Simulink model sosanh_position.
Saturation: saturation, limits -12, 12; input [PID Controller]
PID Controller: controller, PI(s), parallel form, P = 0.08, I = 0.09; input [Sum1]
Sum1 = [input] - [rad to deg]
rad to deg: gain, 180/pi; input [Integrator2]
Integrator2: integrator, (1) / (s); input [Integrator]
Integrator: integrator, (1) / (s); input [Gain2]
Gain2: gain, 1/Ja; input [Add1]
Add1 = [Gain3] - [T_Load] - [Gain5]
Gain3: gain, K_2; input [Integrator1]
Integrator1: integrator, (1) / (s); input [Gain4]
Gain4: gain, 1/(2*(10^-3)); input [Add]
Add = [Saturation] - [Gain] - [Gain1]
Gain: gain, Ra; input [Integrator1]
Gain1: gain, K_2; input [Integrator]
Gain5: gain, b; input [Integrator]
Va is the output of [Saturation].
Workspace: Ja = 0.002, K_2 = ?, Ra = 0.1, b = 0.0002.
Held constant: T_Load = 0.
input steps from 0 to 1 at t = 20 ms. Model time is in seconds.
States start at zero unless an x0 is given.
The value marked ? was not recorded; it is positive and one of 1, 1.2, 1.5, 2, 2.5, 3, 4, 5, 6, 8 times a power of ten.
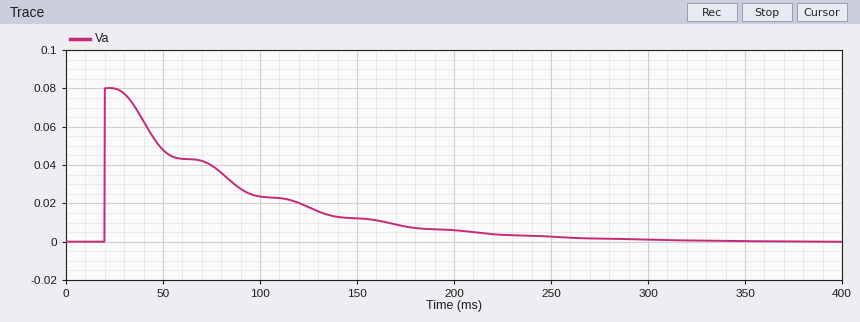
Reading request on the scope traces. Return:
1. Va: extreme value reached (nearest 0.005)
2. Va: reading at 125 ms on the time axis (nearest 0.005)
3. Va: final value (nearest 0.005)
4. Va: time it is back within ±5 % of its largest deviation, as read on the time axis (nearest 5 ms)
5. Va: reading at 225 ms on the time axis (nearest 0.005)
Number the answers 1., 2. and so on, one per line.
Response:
1. 0.080
2. 0.020
3. 0.000
4. 220 ms
5. 0.005
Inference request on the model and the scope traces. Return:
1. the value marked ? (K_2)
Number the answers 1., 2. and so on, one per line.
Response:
1. 0.3
